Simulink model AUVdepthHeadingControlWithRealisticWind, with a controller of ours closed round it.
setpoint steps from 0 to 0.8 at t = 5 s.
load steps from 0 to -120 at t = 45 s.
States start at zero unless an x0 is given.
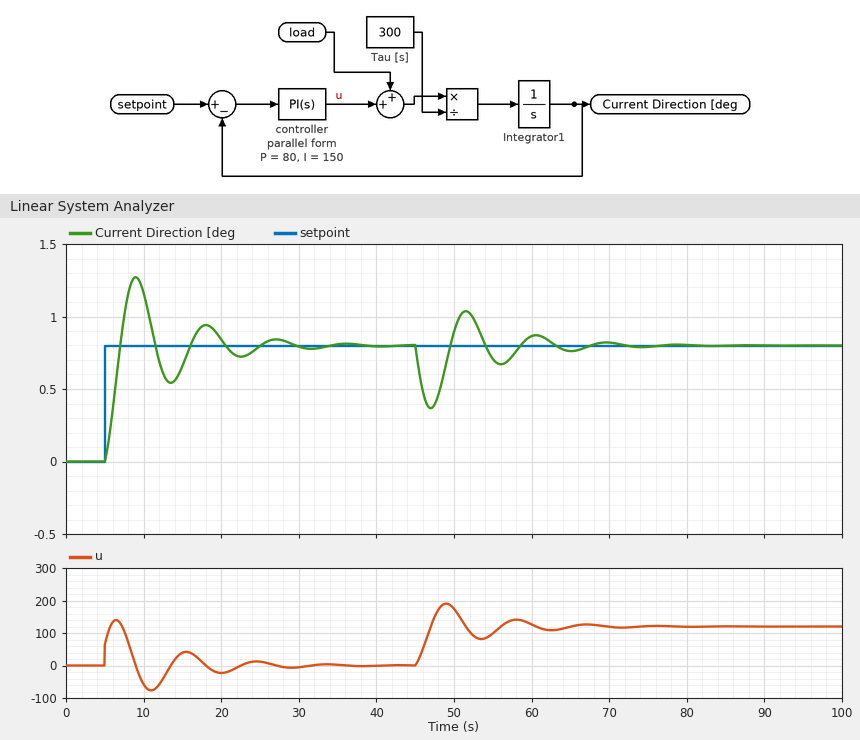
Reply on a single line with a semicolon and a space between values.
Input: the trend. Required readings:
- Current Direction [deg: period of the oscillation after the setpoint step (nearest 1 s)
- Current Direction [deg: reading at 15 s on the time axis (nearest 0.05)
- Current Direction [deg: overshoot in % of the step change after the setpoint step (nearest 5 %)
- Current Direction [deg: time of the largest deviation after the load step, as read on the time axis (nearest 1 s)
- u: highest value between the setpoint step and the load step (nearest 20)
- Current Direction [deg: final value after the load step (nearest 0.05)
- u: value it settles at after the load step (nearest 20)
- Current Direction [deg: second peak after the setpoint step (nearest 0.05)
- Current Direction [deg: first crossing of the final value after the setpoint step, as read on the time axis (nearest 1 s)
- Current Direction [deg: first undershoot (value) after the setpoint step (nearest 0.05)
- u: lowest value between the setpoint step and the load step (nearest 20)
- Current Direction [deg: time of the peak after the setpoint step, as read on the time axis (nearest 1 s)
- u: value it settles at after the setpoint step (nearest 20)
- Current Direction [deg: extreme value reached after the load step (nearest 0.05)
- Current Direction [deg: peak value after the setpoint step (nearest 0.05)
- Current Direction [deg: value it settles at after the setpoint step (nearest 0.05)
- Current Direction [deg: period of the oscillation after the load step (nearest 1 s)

9 s; 0.65; 60 %; 47 s; 140; 0.80; 120; 0.95; 7 s; 0.55; -80; 9 s; 0; 0.35; 1.25; 0.80; 9 s
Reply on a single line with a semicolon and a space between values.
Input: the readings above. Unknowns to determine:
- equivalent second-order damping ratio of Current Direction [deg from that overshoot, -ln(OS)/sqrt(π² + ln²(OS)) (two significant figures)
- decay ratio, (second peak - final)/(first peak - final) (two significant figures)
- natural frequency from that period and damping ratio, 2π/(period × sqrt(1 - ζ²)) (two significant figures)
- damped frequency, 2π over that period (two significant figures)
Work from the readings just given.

0.16; 0.33; 0.71 rad/s; 0.70 rad/s
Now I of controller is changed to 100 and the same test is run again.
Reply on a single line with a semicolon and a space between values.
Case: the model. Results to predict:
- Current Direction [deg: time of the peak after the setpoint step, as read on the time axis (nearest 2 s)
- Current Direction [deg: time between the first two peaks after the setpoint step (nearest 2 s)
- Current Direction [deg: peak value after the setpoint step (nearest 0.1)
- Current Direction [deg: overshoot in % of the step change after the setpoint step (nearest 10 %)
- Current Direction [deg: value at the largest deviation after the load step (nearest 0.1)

10 s; 12 s; 1.2; 50 %; 0.3
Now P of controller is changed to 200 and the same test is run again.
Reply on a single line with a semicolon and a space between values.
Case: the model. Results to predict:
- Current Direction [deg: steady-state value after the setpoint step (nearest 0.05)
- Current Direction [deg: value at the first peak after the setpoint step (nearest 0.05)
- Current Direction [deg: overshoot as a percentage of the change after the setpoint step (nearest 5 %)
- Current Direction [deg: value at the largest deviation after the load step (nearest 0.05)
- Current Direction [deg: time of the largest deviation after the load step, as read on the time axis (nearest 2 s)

0.80; 1.05; 30 %; 0.50; 46 s
